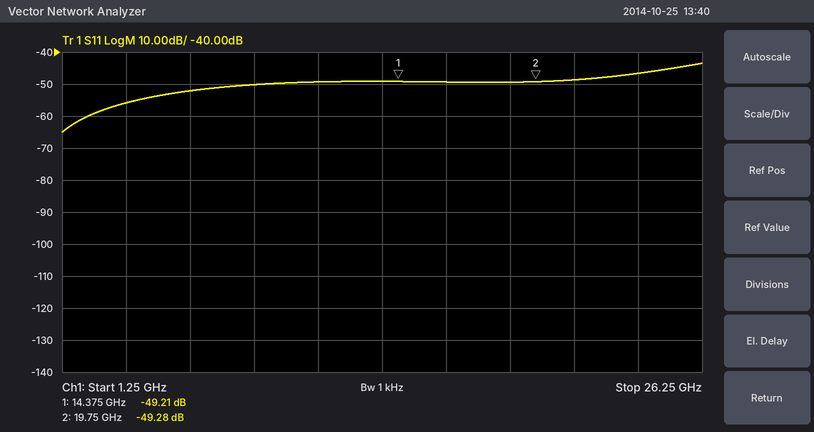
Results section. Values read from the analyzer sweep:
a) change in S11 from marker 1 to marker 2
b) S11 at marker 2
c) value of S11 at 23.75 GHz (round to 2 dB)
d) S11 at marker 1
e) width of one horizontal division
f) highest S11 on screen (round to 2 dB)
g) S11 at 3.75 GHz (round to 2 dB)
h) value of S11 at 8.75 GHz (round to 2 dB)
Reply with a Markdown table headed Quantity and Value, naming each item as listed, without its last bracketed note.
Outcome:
| Quantity | Value |
|---|---|
| change in S11 from marker 1 to marker 2 | -0.07 dB |
| S11 at marker 2 | -49.28 dB |
| value of S11 at 23.75 GHz | -46 dB |
| S11 at marker 1 | -49.21 dB |
| width of one horizontal division | 2.5 GHz |
| highest S11 on screen | -44 dB |
| S11 at 3.75 GHz | -56 dB |
| value of S11 at 8.75 GHz | -50 dB |
